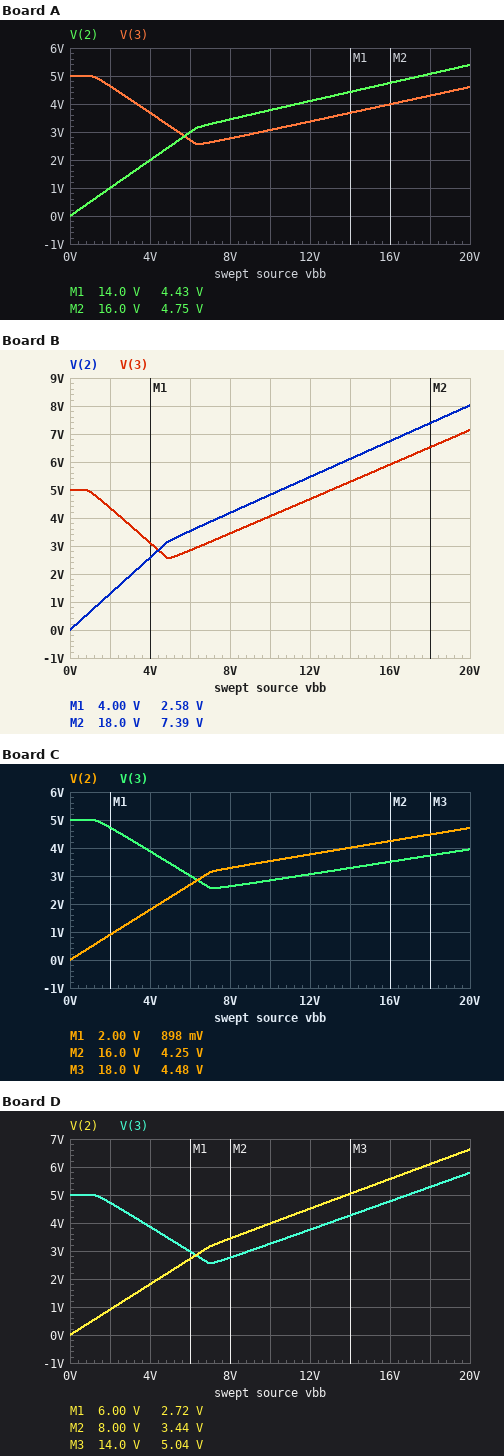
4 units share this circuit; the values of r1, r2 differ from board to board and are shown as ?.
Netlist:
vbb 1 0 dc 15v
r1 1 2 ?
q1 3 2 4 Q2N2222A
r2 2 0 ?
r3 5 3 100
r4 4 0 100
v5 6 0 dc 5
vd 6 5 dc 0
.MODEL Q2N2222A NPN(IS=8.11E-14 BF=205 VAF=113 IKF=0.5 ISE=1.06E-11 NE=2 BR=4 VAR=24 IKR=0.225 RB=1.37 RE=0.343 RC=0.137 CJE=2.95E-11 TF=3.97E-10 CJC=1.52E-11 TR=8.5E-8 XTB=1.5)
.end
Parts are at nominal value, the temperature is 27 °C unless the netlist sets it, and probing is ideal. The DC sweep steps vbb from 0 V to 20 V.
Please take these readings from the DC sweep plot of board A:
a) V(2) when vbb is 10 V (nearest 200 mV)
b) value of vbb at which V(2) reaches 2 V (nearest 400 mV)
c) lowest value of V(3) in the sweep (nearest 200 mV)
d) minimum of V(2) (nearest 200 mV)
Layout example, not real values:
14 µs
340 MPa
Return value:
3.8 V
4.0 V
2.6 V
0 V
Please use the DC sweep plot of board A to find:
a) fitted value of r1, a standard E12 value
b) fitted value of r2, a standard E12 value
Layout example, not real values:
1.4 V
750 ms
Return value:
220 Ω
220 Ω
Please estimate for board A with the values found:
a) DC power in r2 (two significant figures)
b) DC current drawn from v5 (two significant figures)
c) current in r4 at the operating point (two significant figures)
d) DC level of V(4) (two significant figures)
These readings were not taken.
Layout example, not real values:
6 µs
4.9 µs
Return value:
96 mW
12 mA
38 mA
3.8 V
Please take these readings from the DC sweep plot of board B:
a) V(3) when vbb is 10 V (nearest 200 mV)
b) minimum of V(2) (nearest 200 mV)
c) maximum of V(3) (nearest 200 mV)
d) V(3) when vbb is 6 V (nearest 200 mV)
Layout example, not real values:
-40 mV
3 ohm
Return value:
4.0 V
0 V
7.2 V
2.8 V
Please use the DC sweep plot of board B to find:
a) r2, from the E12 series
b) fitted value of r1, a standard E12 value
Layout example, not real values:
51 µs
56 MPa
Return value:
150 Ω
82 Ω
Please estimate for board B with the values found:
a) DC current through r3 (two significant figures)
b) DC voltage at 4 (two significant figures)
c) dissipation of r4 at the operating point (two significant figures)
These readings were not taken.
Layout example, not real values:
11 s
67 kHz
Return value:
6.0 mA
5.6 V
310 mW
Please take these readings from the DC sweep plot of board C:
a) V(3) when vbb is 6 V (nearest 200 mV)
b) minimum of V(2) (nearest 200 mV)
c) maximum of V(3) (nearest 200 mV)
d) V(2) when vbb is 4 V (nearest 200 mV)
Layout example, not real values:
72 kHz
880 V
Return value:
3.0 V
0 V
5.0 V
1.8 V
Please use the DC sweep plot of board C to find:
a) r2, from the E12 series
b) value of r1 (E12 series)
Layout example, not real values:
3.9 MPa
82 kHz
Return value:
270 Ω
330 Ω
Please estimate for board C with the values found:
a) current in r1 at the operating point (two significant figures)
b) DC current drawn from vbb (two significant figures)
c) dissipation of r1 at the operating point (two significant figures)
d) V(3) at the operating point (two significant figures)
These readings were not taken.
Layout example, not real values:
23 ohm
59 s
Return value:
33 mA
33 mA
360 mW
3.4 V
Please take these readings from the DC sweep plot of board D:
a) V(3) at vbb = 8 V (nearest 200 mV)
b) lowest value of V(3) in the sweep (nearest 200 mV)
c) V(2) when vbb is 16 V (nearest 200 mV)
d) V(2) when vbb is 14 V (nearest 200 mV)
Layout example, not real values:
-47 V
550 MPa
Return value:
2.8 V
2.6 V
5.6 V
5.0 V
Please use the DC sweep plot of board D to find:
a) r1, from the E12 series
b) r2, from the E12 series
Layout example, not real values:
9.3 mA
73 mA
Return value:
82 Ω
68 Ω
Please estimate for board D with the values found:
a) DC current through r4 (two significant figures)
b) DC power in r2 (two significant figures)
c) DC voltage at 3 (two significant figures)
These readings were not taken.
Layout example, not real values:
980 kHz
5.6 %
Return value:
45 mA
410 mW
4.5 V
